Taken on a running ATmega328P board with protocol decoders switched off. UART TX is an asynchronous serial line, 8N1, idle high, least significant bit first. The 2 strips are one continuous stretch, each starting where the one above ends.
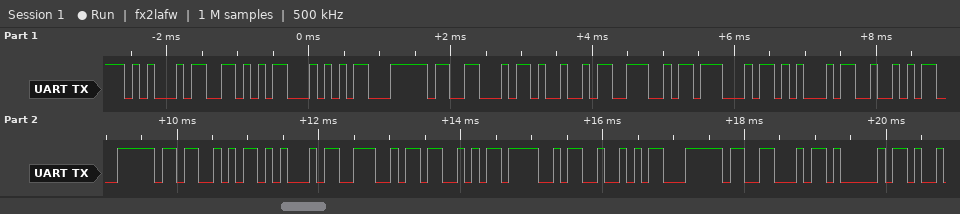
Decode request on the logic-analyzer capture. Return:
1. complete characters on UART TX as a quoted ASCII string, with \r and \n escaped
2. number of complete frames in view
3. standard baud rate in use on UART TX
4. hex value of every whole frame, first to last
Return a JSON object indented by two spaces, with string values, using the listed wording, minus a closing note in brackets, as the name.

{
  "complete characters on UART TX as a quoted ASCII string, with \\r and \\n escaped": "\"EVT|FINGER|SENSOR|FA\"",
  "number of complete frames in view": "20",
  "standard baud rate in use on UART TX": "9600 baud",
  "hex value of every whole frame, first to last": "0x45 0x56 0x54 0x7C 0x46 0x49 0x4E 0x47 0x45 0x52 0x7C 0x53 0x45 0x4E 0x53 0x4F 0x52 0x7C 0x46 0x41"
}
